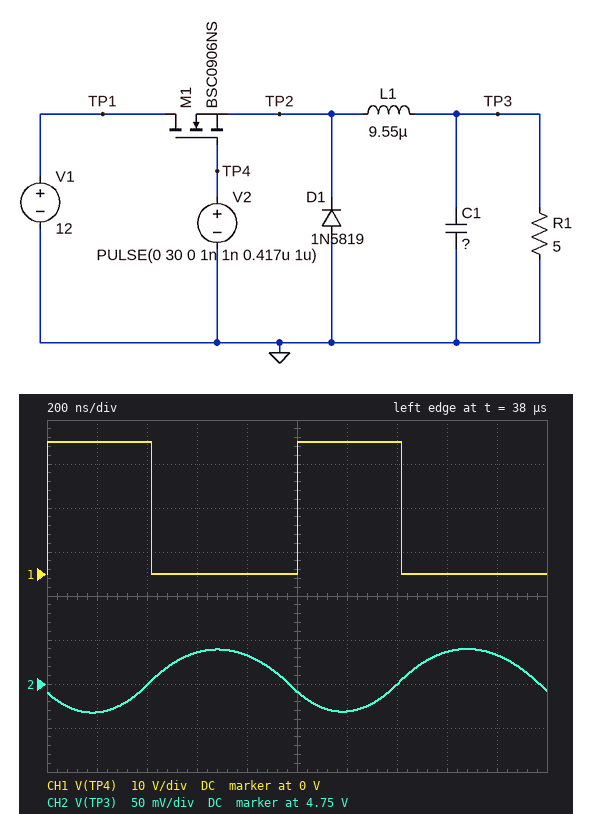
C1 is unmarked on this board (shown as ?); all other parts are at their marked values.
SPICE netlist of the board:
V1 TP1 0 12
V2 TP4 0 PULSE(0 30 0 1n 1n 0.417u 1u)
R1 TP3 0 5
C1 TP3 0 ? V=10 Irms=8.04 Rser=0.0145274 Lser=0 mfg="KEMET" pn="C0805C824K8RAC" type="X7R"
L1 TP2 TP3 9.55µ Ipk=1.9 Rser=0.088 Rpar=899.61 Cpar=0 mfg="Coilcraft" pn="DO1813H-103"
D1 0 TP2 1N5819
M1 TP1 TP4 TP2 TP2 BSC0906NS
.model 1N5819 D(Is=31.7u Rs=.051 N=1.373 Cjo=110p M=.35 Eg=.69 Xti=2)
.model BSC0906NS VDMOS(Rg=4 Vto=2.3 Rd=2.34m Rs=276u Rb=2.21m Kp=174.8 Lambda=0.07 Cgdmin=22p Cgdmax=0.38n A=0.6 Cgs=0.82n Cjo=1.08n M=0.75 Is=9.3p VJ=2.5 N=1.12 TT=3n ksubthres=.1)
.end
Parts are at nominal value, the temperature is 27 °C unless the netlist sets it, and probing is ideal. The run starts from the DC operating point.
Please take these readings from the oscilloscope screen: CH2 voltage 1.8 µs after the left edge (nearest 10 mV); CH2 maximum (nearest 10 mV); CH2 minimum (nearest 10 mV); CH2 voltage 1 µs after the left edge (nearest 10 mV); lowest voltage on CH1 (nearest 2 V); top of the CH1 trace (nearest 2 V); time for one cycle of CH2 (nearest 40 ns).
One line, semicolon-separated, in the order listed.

4.78 V; 4.79 V; 4.72 V; 4.74 V; 0 V; 30 V; 1.00 µs
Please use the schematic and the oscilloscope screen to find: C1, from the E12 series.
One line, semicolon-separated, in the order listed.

560 nF
